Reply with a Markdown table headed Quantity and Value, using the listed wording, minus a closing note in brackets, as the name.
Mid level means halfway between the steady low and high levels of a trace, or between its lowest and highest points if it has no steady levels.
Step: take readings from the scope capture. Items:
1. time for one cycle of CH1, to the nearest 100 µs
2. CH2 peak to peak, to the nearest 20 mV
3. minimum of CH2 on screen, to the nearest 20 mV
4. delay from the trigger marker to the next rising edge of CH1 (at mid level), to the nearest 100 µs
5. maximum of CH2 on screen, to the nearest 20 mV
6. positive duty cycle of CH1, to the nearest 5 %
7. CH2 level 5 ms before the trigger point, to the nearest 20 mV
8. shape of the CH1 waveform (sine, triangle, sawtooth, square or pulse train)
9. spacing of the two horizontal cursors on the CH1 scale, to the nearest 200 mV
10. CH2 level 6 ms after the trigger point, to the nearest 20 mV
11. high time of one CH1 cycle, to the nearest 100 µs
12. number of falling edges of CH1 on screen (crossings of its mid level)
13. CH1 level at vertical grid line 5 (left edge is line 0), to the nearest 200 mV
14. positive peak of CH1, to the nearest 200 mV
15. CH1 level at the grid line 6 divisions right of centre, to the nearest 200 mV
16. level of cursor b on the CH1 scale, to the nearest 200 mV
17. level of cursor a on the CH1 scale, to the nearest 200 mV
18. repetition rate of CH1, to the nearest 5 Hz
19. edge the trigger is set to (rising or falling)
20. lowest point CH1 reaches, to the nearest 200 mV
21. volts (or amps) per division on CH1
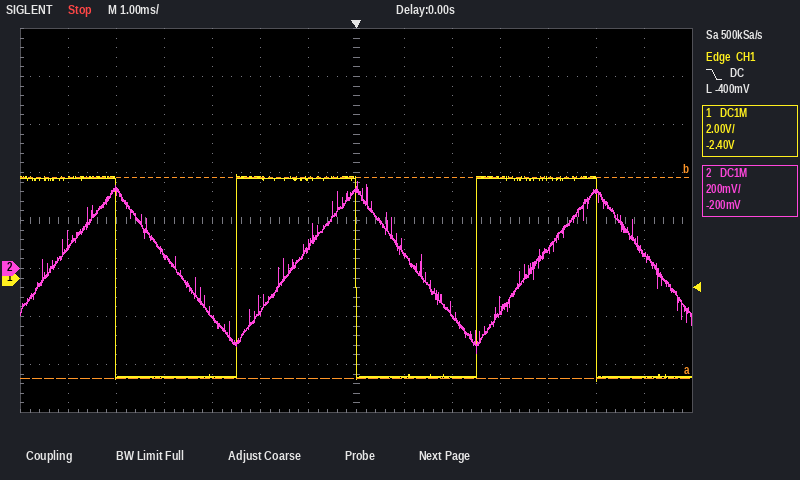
| Quantity | Value |
|---|---|
| time for one cycle of CH1, to the nearest 100 µs | 5.0 ms |
| CH2 peak to peak, to the nearest 20 mV | 720 mV |
| minimum of CH2 on screen, to the nearest 20 mV | -360 mV |
| delay from the trigger marker to the next rising edge of CH1 (at mid level), to the nearest 100 µs | 2.5 ms |
| maximum of CH2 on screen, to the nearest 20 mV | 360 mV |
| positive duty cycle of CH1, to the nearest 5 % | 50 % |
| CH2 level 5 ms before the trigger point, to the nearest 20 mV | 320 mV |
| shape of the CH1 waveform | square |
| spacing of the two horizontal cursors on the CH1 scale, to the nearest 200 mV | 8.4 V |
| CH2 level 6 ms after the trigger point, to the nearest 20 mV | 60 mV |
| high time of one CH1 cycle, to the nearest 100 µs | 2.5 ms |
| number of falling edges of CH1 on screen | 3 |
| CH1 level at vertical grid line 5 (left edge is line 0), to the nearest 200 mV | 4.2 V |
| positive peak of CH1, to the nearest 200 mV | 4.4 V |
| CH1 level at the grid line 6 divisions right of centre, to the nearest 200 mV | -4.2 V |
| level of cursor b on the CH1 scale, to the nearest 200 mV | 4.2 V |
| level of cursor a on the CH1 scale, to the nearest 200 mV | -4.2 V |
| repetition rate of CH1, to the nearest 5 Hz | 200 Hz |
| edge the trigger is set to | falling |
| lowest point CH1 reaches, to the nearest 200 mV | -4.4 V |
| volts (or amps) per division on CH1 | 2 V |
